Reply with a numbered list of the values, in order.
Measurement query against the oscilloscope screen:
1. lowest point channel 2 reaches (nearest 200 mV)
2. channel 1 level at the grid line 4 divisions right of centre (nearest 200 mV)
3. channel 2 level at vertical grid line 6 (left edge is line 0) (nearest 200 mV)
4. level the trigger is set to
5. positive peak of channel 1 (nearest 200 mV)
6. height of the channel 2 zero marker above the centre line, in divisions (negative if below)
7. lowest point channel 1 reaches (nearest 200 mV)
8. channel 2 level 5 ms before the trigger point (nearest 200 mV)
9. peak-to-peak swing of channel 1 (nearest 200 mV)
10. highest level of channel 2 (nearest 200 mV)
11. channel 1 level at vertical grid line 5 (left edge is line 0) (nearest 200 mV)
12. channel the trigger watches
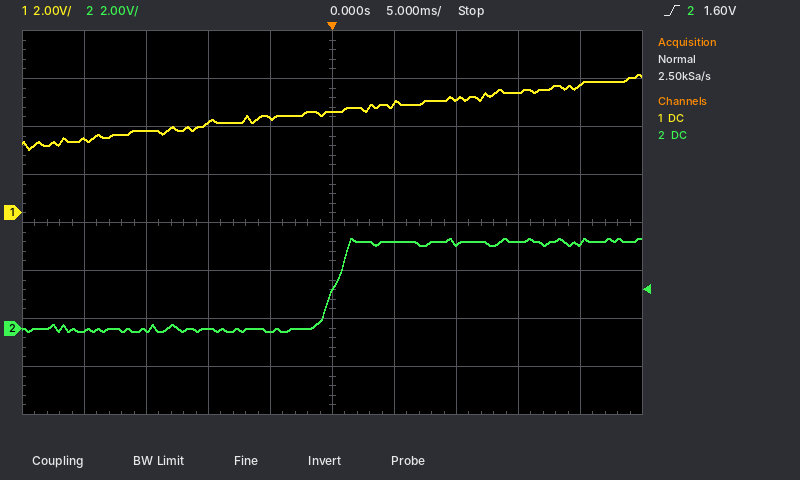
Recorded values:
1. -200 mV
2. 5.4 V
3. 3.6 V
4. 1.60 V
5. 5.8 V
6. -2.2 div
7. 2.6 V
8. -200 mV
9. 3.2 V
10. 3.8 V
11. 4.2 V
12. channel 2
